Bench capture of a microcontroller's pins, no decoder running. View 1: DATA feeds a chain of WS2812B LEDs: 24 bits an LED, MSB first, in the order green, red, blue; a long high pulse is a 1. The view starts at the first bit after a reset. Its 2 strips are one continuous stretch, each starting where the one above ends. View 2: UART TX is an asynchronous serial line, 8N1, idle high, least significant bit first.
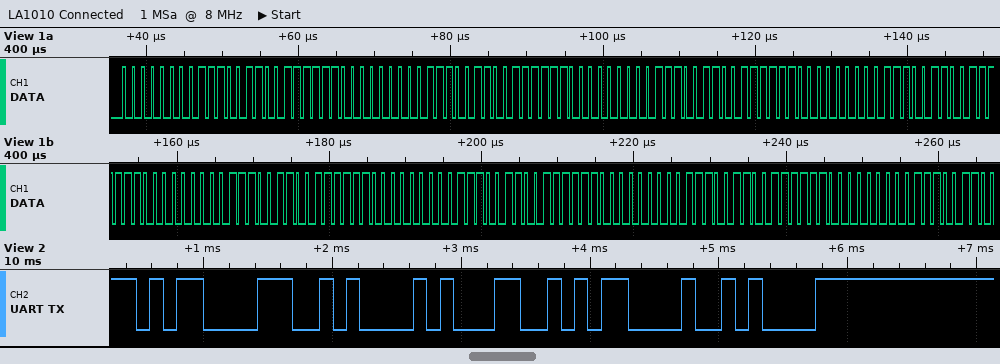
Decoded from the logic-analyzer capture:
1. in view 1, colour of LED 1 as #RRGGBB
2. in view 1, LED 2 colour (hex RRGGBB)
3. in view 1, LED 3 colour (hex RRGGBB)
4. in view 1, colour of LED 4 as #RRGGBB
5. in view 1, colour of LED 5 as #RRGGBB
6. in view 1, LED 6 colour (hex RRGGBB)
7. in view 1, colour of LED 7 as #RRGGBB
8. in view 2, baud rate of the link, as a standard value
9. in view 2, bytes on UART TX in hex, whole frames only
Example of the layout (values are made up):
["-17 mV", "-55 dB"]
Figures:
["#E6007E", "#E6007E", "#E6007E", "#E6007E", "#E6007E", "#E6007E", "#E6007E", "9600 baud", "0D 0A 31 0D 0A"]
